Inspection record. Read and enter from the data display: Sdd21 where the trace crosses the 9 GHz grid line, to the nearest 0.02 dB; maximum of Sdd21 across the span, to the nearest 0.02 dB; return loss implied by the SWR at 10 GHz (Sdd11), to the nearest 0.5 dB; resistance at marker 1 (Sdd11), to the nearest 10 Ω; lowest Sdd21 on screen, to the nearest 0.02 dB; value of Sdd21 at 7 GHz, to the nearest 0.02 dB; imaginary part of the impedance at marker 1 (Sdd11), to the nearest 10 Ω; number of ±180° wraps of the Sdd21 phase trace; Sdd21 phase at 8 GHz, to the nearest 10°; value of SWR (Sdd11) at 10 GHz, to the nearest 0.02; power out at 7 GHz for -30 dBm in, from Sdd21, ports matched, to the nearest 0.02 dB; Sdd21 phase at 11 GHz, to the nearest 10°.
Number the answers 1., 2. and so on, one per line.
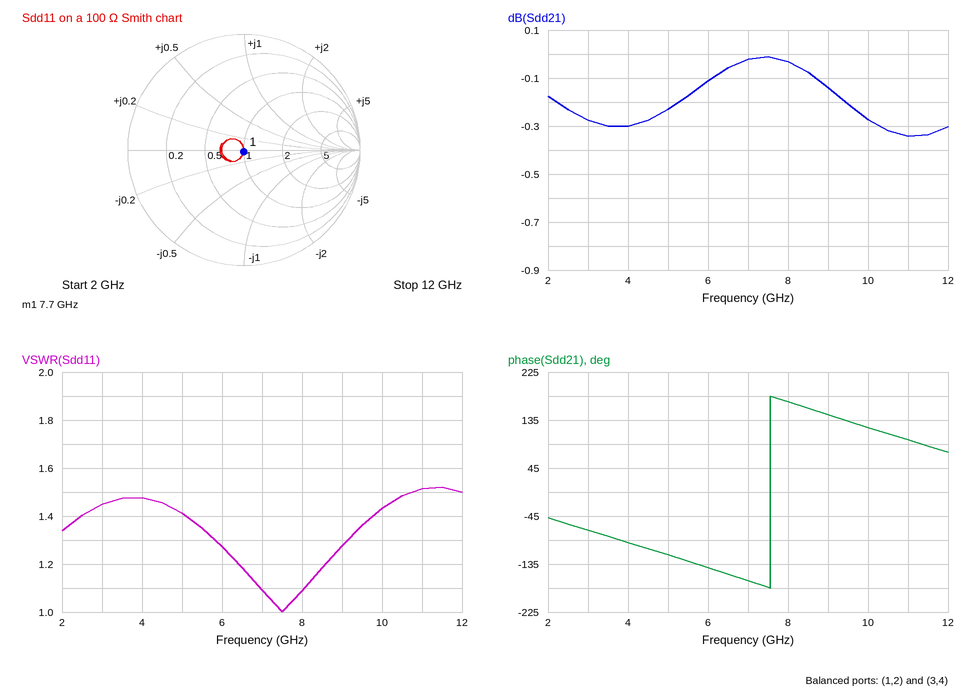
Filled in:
1. -0.14 dB
2. -0.02 dB
3. 15.0 dB
4. 100 Ω
5. -0.34 dB
6. -0.02 dB
7. 0 Ω
8. 1
9. 170°
10. 1.44
11. -30.02 dBm
12. 100°
